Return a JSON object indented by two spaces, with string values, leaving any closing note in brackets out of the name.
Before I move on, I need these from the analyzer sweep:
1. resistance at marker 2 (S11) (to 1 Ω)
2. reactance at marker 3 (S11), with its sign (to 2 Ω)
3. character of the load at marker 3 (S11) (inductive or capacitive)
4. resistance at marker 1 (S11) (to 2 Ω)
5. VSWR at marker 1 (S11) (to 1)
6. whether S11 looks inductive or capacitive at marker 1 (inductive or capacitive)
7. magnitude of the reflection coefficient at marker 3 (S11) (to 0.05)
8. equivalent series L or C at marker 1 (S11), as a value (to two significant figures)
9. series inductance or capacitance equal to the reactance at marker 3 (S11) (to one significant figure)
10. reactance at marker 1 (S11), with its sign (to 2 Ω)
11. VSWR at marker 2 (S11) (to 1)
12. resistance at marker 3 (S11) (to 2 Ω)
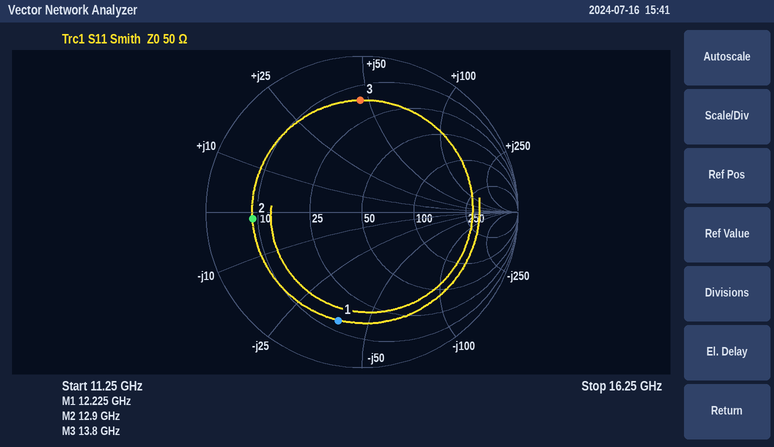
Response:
{
  "resistance at marker 2 (S11)": "9 Ω",
  "reactance at marker 3 (S11), with its sign": "+46 Ω",
  "character of the load at marker 3 (S11)": "inductive",
  "resistance at marker 1 (S11)": "14 Ω",
  "VSWR at marker 1 (S11)": "6",
  "whether S11 looks inductive or capacitive at marker 1": "capacitive",
  "magnitude of the reflection coefficient at marker 3 (S11)": "0.70",
  "equivalent series L or C at marker 1 (S11), as a value": "340 fF",
  "series inductance or capacitance equal to the reactance at marker 3 (S11)": "500 pH",
  "reactance at marker 1 (S11), with its sign": "-38 Ω",
  "VSWR at marker 2 (S11)": "6",
  "resistance at marker 3 (S11)": "16 Ω"
}
